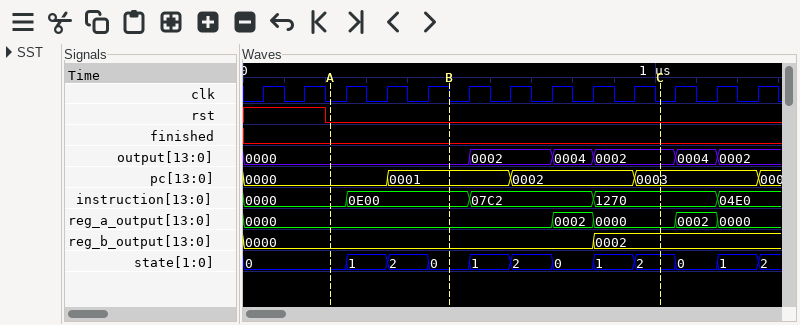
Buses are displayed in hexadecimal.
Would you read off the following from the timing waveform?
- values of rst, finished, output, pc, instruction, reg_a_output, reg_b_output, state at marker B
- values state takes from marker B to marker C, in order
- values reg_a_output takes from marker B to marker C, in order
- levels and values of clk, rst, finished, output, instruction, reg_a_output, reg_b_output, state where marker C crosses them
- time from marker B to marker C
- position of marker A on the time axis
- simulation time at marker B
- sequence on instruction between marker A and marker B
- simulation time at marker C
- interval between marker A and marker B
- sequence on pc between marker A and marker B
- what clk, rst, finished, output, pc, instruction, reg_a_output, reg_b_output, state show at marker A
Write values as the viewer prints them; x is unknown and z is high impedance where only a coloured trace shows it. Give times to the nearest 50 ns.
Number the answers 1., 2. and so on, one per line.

1. rst=0, finished=0, output=0000, pc=0001, instruction=0E00, reg_a_output=0000, reg_b_output=0000, state=0
2. 0, 1, 2, 0, 1, 2
3. 0000, 0002, 0000
4. clk=0, rst=0, finished=0, output=0002, instruction=1270, reg_a_output=0000, reg_b_output=0002, state=2
5. 500 ns
6. 200 ns
7. 500 ns
8. 0000, 0E00
9. 1000 ns
10. 300 ns
11. 0000, 0001
12. clk=0, rst=0, finished=0, output=0000, pc=0000, instruction=0000, reg_a_output=0000, reg_b_output=0000, state=0
